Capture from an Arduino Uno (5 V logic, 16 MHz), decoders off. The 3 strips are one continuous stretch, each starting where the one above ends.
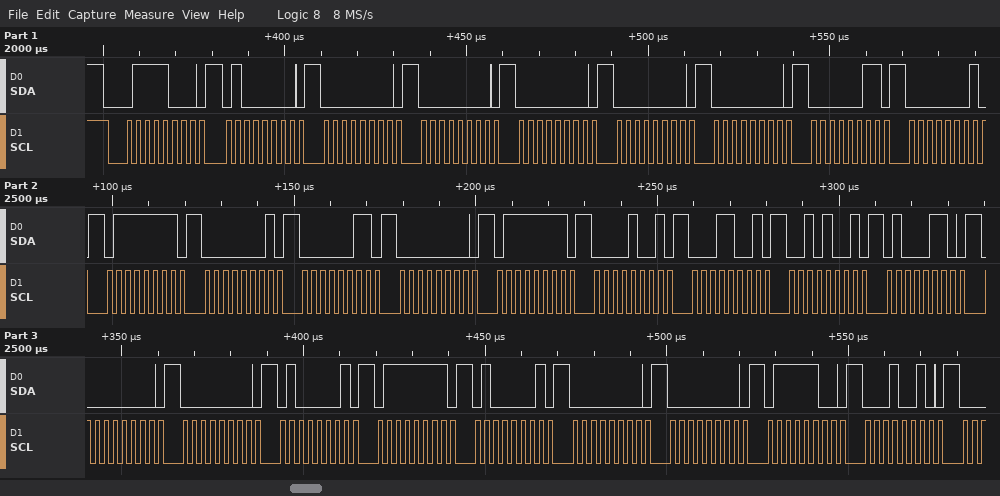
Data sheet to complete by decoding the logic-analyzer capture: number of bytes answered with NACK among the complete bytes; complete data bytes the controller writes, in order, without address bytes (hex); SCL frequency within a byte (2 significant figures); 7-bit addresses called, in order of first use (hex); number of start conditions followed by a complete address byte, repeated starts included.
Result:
0
40 00 00 00 00 00 03 01 7F 01 03 00 7F 09 19 29 46 00 00 41 7F 41 00 00 7C 12
400 kHz
0x3C
1
